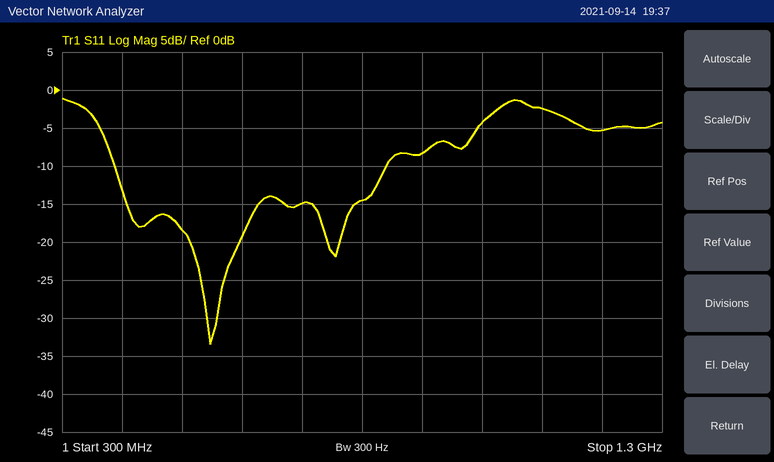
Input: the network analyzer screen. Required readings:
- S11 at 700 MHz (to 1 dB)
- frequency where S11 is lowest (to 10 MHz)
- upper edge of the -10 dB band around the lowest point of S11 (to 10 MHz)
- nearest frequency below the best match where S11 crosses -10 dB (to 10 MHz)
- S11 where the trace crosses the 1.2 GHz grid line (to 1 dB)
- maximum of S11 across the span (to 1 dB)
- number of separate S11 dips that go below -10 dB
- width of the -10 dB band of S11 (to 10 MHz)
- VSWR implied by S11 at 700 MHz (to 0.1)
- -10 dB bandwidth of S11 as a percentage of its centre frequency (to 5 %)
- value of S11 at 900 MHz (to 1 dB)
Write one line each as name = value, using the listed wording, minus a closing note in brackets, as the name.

S11 at 700 MHz = -15 dB
frequency where S11 is lowest = 550 MHz
upper edge of the -10 dB band around the lowest point of S11 = 840 MHz
nearest frequency below the best match where S11 crosses -10 dB = 390 MHz
S11 where the trace crosses the 1.2 GHz grid line = -5 dB
maximum of S11 across the span = -1 dB
number of separate S11 dips that go below -10 dB = 2
width of the -10 dB band of S11 = 450 MHz
VSWR implied by S11 at 700 MHz = 1.4
-10 dB bandwidth of S11 as a percentage of its centre frequency = 75 %
value of S11 at 900 MHz = -8 dB
